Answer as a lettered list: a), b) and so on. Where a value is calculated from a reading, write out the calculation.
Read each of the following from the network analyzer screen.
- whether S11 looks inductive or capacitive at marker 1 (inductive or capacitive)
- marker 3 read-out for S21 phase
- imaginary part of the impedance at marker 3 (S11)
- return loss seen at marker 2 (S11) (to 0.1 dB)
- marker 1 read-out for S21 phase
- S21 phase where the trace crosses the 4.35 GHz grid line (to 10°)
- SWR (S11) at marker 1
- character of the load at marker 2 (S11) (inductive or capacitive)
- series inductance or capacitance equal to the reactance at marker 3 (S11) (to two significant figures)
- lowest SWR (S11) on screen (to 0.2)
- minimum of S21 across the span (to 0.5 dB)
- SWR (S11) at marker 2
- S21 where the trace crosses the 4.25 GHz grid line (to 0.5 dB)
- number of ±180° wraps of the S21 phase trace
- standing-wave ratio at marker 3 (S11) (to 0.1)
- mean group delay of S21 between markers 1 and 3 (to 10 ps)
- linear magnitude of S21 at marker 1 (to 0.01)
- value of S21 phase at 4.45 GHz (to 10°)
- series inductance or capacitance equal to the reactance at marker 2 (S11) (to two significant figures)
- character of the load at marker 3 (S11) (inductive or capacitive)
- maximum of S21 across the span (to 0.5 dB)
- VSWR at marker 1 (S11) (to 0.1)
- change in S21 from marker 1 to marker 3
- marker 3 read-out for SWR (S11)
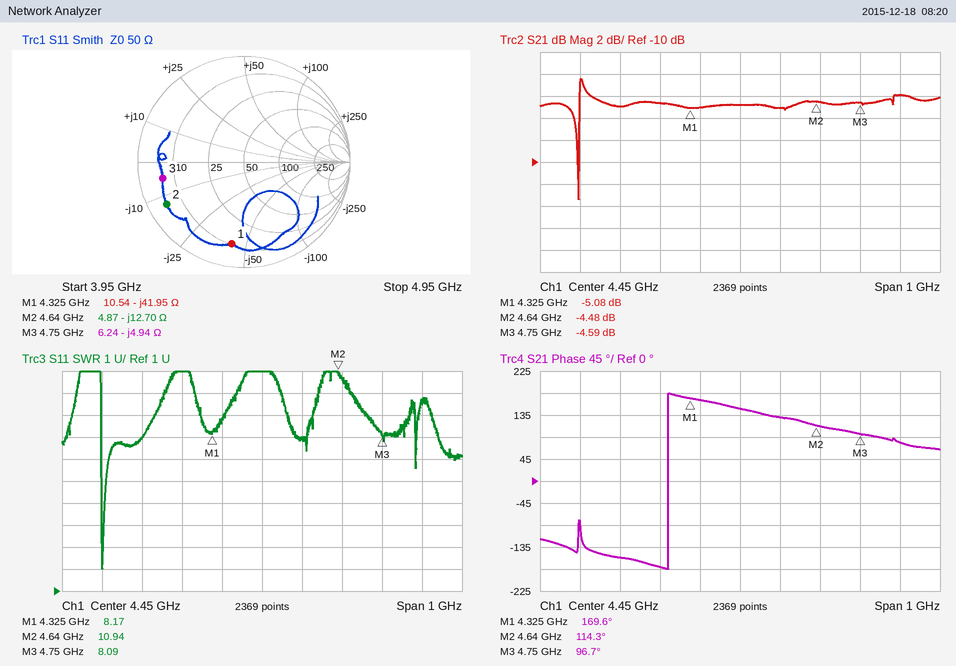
a) capacitive
b) 96.7°
c) -4.94 Ω
d) 1.6 dB
e) 169.6°
f) 170°
g) 8.17
h) capacitive
i) C = 1/(2π × 4.75 GHz × 4.94 Ω) ≈ 6.8 pF
j) 2.0
k) -13.5 dB
l) 10.94
m) -4.5 dB
n) 1
o) 8.1
p) −(96.7° − (169.6°))/(360° × 425 MHz) ≈ 476 ps, so 480 ps to the nearest 10 ps
q) 10^(-5.08/20) ≈ 0.56
r) 150°
s) C = 1/(2π × 4.64 GHz × 12.7 Ω) ≈ 2.7 pF
t) capacitive
u) -2.5 dB
v) 8.2
w) -4.59 − (-5.08) = 0.49 dB
x) 8.09
